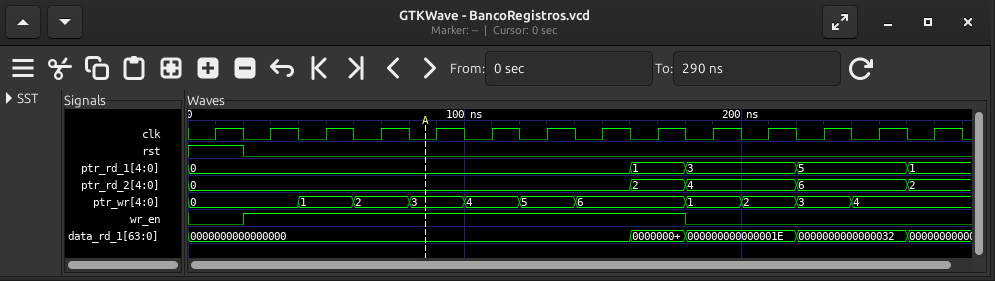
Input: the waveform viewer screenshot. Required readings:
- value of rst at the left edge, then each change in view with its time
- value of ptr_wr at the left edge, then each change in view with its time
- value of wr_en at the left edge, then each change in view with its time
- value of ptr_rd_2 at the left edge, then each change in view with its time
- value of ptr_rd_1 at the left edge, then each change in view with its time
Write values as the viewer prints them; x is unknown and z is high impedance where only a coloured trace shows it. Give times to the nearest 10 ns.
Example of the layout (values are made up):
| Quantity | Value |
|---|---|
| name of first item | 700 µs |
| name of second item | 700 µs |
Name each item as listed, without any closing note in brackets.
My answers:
| Quantity | Value |
|---|---|
| value of rst at the left edge, then each change in view with its time | 1, 0 at 20 ns |
| value of ptr_wr at the left edge, then each change in view with its time | 0, 1 at 40 ns, 2 at 60 ns, 3 at 80 ns, 4 at 100 ns, 5 at 120 ns, 6 at 140 ns, 1 at 180 ns, 2 at 200 ns, 3 at 220 ns, 4 at 240 ns |
| value of wr_en at the left edge, then each change in view with its time | 0, 1 at 20 ns, 0 at 180 ns |
| value of ptr_rd_2 at the left edge, then each change in view with its time | 0, 2 at 160 ns, 4 at 180 ns, 6 at 220 ns, 2 at 260 ns |
| value of ptr_rd_1 at the left edge, then each change in view with its time | 0, 1 at 160 ns, 3 at 180 ns, 5 at 220 ns, 1 at 260 ns |
